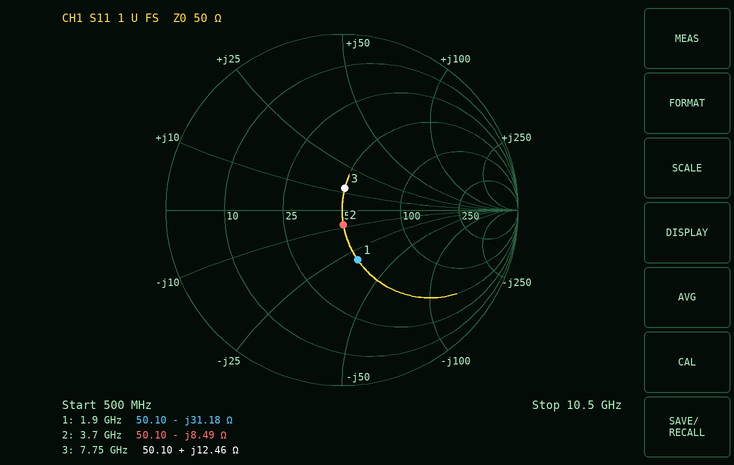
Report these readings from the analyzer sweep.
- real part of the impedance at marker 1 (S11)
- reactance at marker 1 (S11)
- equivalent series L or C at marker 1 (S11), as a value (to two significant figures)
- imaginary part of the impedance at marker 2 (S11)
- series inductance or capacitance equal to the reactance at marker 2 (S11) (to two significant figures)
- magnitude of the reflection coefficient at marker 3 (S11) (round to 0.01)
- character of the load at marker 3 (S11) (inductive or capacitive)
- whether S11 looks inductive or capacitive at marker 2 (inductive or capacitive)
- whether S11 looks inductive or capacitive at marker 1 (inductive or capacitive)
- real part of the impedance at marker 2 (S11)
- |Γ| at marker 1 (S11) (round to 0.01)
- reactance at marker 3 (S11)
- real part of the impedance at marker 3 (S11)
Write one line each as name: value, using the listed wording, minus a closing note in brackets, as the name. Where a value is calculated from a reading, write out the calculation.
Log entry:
real part of the impedance at marker 1: 50.10 Ω
reactance at marker 1: -31.18 Ω
equivalent series L or C at marker 1 (S11), as a value: C = 1/(2π × 1.9 GHz × 31.18 Ω) ≈ 2.7 pF
imaginary part of the impedance at marker 2: -8.49 Ω
series inductance or capacitance equal to the reactance at marker 2 (S11): C = 1/(2π × 3.7 GHz × 8.49 Ω) ≈ 5.1 pF
magnitude of the reflection coefficient at marker 3 (S11): 0.12
character of the load at marker 3 (S11): inductive
whether S11 looks inductive or capacitive at marker 2: capacitive
whether S11 looks inductive or capacitive at marker 1: capacitive
real part of the impedance at marker 2: 50.10 Ω
|Γ| at marker 1 (S11): 0.30
reactance at marker 3: +12.46 Ω
real part of the impedance at marker 3: 50.10 Ω
